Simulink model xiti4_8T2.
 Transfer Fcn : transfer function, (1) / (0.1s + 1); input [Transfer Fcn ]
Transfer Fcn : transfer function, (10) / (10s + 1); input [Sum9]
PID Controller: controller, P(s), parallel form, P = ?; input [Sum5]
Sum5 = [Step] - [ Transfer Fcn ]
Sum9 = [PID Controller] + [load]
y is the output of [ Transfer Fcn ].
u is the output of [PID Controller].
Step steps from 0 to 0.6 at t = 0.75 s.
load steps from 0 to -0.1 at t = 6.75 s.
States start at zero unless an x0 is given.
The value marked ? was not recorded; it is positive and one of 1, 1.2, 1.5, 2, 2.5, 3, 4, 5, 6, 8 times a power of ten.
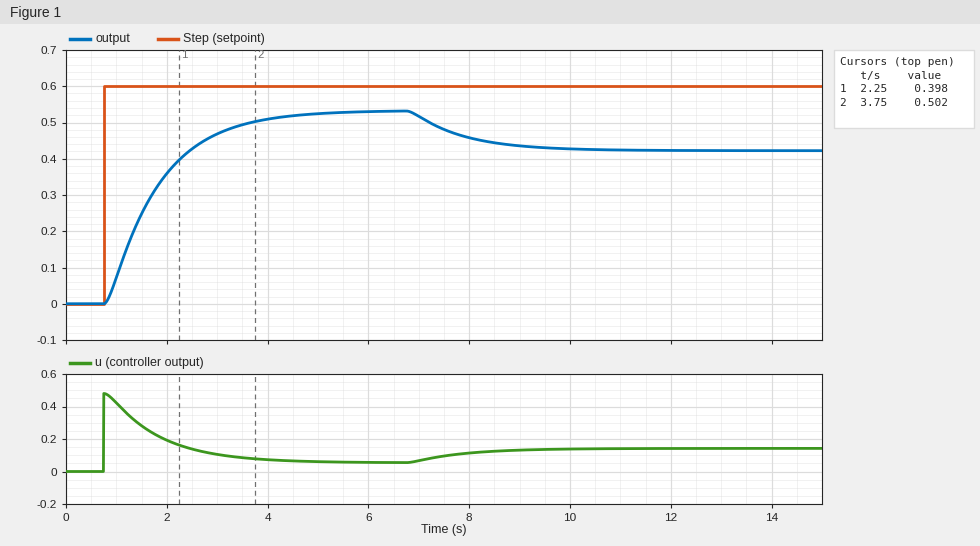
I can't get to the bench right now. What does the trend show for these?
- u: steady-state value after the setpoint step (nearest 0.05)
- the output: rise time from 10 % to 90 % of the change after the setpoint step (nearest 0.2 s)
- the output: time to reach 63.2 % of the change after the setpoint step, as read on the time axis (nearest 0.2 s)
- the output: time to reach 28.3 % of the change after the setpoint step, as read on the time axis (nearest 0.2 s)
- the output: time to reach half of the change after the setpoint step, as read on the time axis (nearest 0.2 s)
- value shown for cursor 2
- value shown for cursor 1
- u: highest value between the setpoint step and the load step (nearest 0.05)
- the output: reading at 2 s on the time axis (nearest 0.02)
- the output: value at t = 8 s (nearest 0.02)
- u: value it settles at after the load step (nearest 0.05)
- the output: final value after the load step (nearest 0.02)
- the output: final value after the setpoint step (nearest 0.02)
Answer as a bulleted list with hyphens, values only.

- 0.05
- 2.2 s
- 1.8 s
- 1.2 s
- 1.6 s
- 0.502
- 0.398
- 0.50
- 0.36
- 0.46
- 0.15
- 0.42
- 0.54
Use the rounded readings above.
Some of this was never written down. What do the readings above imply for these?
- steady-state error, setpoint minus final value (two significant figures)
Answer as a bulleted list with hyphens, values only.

- 0.060
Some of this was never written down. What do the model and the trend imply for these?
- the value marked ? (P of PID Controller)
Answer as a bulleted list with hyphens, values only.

- 0.8
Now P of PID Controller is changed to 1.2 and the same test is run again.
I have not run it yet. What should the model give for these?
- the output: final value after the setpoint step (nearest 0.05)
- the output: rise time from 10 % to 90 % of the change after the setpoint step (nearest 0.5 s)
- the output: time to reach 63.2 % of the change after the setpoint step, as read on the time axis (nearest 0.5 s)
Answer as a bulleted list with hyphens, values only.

- 0.55
- 1.5 s
- 1.5 s
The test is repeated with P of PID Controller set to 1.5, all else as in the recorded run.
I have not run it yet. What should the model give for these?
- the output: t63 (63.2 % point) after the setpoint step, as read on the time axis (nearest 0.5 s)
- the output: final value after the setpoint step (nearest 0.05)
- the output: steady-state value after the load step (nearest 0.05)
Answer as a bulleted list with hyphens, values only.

- 1.5 s
- 0.55
- 0.50
